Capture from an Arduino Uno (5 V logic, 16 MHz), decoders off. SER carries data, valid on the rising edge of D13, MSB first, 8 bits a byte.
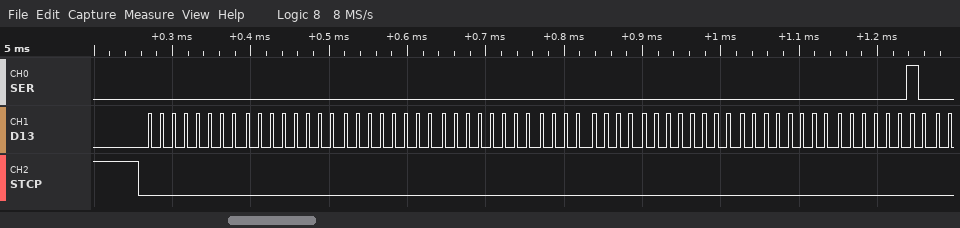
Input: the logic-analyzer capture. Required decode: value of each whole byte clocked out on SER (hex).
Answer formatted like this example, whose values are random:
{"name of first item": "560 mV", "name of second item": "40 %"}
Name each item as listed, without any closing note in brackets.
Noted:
{"value of each whole byte clocked out on SER": "00 00 00 00 00 00 00 02"}
